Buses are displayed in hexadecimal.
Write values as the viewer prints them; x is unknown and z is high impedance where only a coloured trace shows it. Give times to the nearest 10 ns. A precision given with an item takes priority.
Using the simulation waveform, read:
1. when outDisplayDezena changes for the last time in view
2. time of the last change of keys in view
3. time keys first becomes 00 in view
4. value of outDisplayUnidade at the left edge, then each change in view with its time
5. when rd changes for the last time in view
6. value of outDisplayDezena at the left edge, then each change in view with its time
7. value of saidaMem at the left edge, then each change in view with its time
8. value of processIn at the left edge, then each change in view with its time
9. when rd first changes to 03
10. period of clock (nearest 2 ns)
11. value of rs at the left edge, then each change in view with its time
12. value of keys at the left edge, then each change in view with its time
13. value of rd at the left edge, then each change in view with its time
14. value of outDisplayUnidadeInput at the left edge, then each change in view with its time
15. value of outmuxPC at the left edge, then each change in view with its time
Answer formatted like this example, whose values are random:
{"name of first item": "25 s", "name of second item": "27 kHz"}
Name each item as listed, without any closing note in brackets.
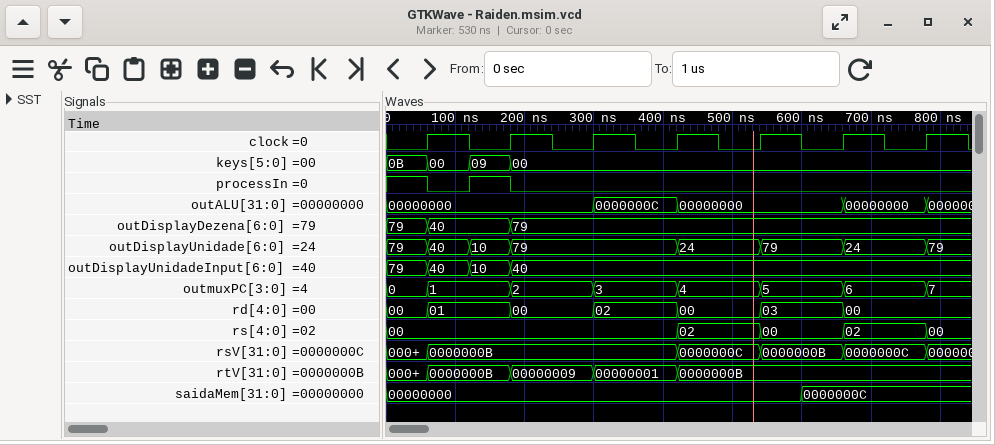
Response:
{"when outDisplayDezena changes for the last time in view": "180 ns", "time of the last change of keys in view": "180 ns", "time keys first becomes 00 in view": "60 ns", "value of outDisplayUnidade at the left edge, then each change in view with its time": "79, 40 at 60 ns, 10 at 120 ns, 79 at 180 ns, 24 at 420 ns, 79 at 540 ns, 24 at 660 ns, 79 at 780 ns", "when rd changes for the last time in view": "660 ns", "value of outDisplayDezena at the left edge, then each change in view with its time": "79, 40 at 60 ns, 79 at 180 ns", "value of saidaMem at the left edge, then each change in view with its time": "00000000, 0000000C at 600 ns", "value of processIn at the left edge, then each change in view with its time": "1, 0 at 60 ns, 1 at 120 ns, 0 at 180 ns", "when rd first changes to 03": "540 ns", "period of clock": "120 ns", "value of rs at the left edge, then each change in view with its time": "00, 02 at 420 ns, 00 at 540 ns, 02 at 660 ns, 00 at 780 ns", "value of keys at the left edge, then each change in view with its time": "0B, 00 at 60 ns, 09 at 120 ns, 00 at 180 ns", "value of rd at the left edge, then each change in view with its time": "00, 01 at 60 ns, 00 at 180 ns, 02 at 300 ns, 00 at 420 ns, 03 at 540 ns, 00 at 660 ns", "value of outDisplayUnidadeInput at the left edge, then each change in view with its time": "79, 40 at 60 ns, 10 at 120 ns, 40 at 180 ns", "value of outmuxPC at the left edge, then each change in view with its time": "0, 1 at 60 ns, 2 at 180 ns, 3 at 300 ns, 4 at 420 ns, 5 at 540 ns, 6 at 660 ns, 7 at 780 ns"}
